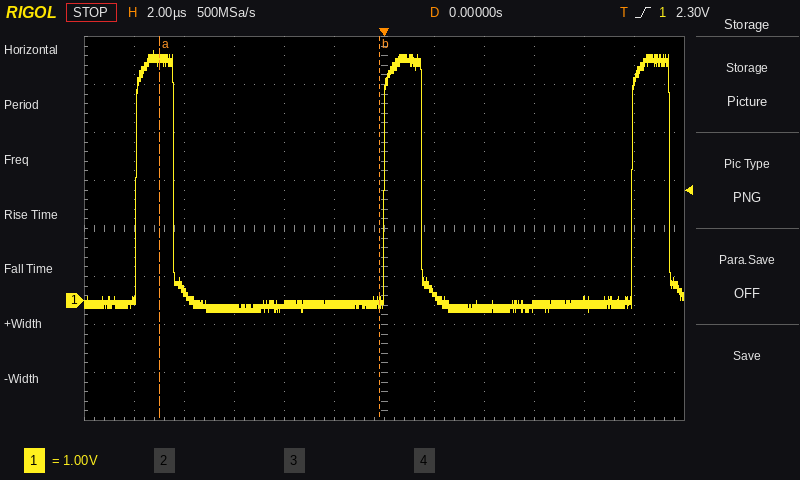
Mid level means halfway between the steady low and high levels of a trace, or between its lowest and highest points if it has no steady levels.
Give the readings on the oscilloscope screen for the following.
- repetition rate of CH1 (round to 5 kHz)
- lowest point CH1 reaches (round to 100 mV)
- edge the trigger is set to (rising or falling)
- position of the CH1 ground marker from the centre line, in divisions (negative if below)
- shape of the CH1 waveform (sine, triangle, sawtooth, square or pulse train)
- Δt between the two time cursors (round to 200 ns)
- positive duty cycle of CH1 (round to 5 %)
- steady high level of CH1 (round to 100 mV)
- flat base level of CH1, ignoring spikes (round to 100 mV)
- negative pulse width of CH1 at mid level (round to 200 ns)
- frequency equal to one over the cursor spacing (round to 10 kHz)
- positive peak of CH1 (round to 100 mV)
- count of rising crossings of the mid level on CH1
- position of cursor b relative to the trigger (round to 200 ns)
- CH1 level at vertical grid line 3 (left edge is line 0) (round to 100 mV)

100 kHz
-200 mV
rising
-1.5 div
pulse train
8.8 µs
15 %
5.0 V
-100 mV
8.4 µs
110 kHz
5.2 V
3
-200 ns
-200 mV
